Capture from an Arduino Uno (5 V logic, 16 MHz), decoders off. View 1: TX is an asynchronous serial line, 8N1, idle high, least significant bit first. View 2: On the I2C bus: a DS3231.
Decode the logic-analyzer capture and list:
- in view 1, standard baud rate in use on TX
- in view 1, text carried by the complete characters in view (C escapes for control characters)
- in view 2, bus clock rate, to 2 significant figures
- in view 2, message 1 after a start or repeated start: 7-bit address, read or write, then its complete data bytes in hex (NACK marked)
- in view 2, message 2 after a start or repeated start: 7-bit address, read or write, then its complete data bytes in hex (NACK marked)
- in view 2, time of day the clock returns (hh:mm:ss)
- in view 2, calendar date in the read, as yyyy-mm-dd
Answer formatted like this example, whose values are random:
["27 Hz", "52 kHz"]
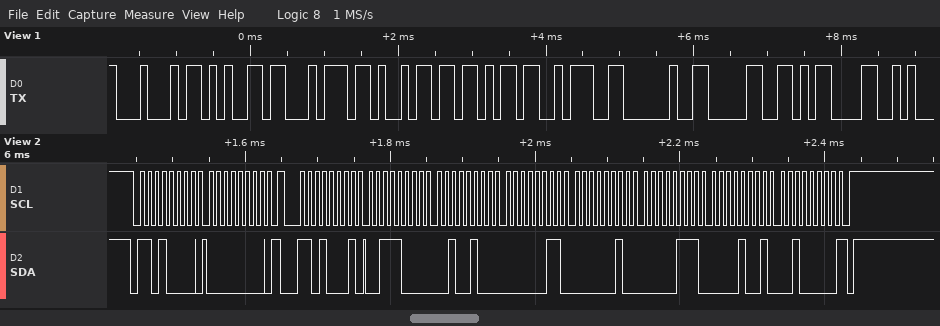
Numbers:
["9600 baud", "\"Detik: 0\\r\"", "100 kHz", "0x68 write: 00", "0x68 read: 38 24 03 02 07 09 20 NACK", "03:24:38", "2020-09-07"]
